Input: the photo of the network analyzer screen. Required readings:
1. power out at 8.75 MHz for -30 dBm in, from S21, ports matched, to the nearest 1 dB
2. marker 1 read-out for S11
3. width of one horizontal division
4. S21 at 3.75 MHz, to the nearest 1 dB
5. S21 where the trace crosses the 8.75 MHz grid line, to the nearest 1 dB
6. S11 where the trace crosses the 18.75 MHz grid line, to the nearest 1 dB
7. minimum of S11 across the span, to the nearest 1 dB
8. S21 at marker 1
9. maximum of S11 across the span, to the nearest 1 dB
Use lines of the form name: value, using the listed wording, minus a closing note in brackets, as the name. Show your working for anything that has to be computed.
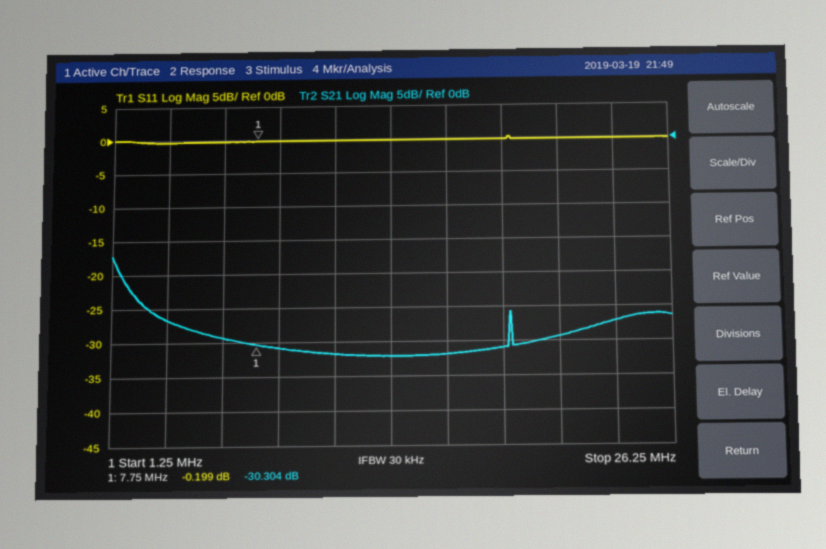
power out at 8.75 MHz for -30 dBm in, from S21, ports matched, to the nearest 1 dB: -30 dBm + (-31 dB) = -61 dBm
marker 1 read-out for S11: -0.199 dB
width of one horizontal division: 2.5 MHz
S21 at 3.75 MHz, to the nearest 1 dB: -27 dB
S21 where the trace crosses the 8.75 MHz grid line, to the nearest 1 dB: -31 dB
S11 where the trace crosses the 18.75 MHz grid line, to the nearest 1 dB: 0 dB
minimum of S11 across the span, to the nearest 1 dB: 0 dB
S21 at marker 1: -30.304 dB
maximum of S11 across the span, to the nearest 1 dB: 0 dB
